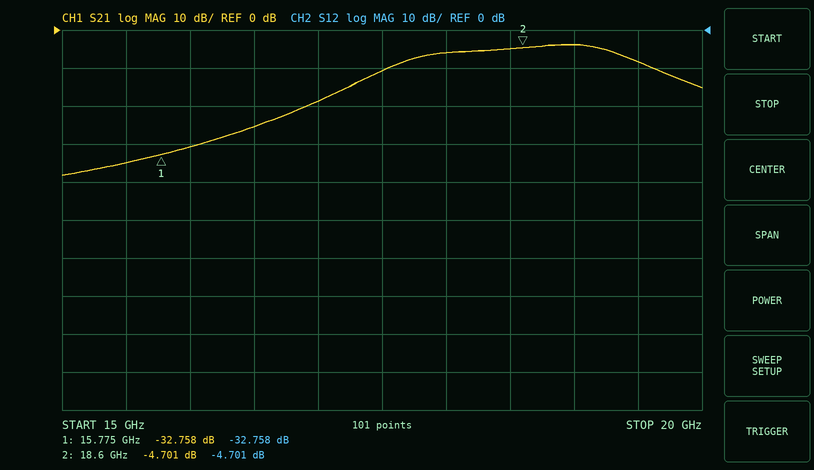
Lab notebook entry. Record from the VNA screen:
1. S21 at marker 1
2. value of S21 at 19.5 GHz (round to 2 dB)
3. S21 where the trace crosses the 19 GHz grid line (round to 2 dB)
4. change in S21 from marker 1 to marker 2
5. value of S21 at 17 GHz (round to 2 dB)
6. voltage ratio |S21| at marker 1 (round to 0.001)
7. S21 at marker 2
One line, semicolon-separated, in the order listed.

-32.758 dB; -8 dB; -4 dB; 28.057 dB; -18 dB; 0.023; -4.701 dB
